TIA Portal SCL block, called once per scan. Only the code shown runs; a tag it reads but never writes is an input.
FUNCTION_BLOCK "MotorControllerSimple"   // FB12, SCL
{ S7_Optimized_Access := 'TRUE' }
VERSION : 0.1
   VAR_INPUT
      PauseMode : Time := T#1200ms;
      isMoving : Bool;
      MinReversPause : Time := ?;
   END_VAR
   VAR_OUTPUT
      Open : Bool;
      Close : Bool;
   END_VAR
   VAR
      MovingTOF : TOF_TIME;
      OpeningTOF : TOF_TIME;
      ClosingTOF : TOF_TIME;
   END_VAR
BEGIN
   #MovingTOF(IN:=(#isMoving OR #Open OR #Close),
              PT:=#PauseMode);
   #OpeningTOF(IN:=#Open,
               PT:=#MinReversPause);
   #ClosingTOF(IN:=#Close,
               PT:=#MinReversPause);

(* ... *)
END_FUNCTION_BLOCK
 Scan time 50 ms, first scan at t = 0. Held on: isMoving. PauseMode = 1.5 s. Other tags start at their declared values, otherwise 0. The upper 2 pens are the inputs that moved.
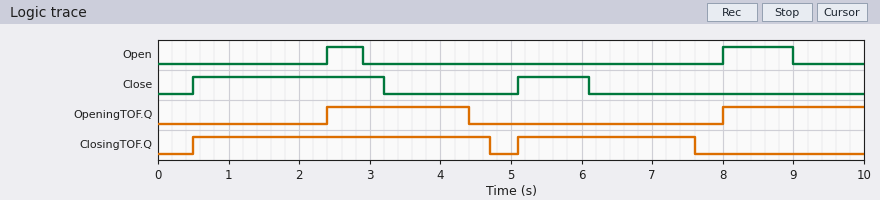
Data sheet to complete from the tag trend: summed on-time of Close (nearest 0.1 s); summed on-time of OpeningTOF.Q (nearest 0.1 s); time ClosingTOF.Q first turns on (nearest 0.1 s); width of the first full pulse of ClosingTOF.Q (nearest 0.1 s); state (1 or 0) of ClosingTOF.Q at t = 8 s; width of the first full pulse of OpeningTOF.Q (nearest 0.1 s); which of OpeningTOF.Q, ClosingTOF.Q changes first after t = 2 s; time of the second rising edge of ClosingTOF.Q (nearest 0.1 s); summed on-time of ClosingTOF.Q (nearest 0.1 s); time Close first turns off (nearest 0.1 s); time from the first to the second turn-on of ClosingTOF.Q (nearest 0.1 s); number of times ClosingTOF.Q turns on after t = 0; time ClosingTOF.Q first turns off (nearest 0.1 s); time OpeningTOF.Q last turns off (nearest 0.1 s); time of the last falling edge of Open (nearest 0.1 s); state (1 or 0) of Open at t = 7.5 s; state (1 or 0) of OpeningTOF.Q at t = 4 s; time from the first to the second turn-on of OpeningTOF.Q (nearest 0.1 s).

3.7 s
4.0 s
0.5 s
4.2 s
0
2.0 s
OpeningTOF.Q
5.1 s
6.7 s
3.2 s
4.6 s
2
4.7 s
4.4 s
9.0 s
0
1
5.6 s
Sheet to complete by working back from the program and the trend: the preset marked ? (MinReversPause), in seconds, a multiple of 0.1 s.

1.5 s
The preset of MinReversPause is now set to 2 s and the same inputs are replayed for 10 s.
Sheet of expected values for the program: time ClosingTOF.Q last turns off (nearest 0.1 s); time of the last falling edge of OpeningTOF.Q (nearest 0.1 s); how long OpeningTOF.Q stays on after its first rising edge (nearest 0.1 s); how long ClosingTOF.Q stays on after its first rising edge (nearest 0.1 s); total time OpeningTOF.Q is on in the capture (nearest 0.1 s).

8.1 s
4.9 s
2.5 s
7.6 s
4.5 s
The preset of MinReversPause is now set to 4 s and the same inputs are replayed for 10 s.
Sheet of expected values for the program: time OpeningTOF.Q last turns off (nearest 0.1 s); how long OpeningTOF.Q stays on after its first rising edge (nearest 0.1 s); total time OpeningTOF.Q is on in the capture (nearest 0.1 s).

6.9 s
4.5 s
6.5 s
